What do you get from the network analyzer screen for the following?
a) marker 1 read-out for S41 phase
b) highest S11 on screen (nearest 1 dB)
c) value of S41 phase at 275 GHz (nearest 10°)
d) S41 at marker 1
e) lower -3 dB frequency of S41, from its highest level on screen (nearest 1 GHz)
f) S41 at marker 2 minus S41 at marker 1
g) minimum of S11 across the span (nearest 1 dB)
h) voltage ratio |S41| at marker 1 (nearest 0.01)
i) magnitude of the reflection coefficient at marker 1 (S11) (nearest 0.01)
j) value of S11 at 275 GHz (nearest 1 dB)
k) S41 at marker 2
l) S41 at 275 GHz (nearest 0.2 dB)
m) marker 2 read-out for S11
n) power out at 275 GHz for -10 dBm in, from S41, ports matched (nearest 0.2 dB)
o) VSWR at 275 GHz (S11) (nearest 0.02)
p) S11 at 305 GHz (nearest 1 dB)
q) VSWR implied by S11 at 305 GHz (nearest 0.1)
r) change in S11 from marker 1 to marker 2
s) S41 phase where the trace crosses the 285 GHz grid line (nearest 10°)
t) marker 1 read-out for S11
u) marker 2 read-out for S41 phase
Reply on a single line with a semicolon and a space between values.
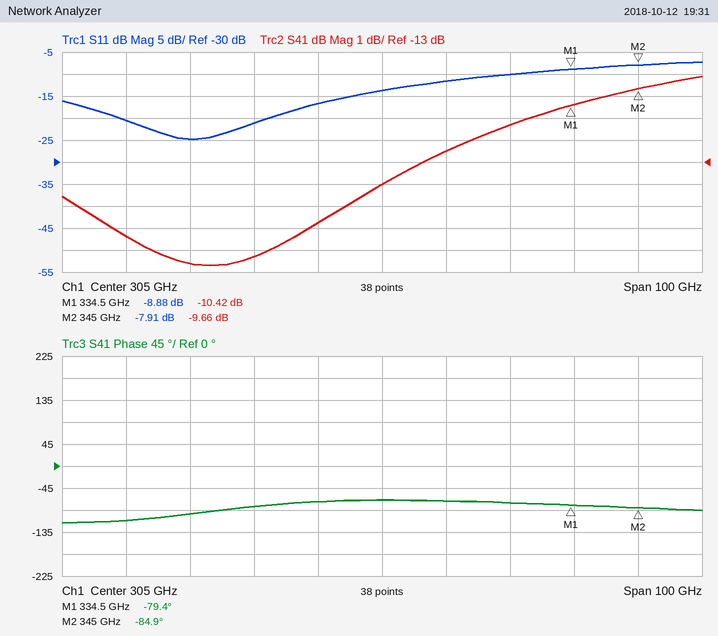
-79.4°; -7 dB; -100°; -10.42 dB; 318 GHz; 0.76 dB; -25 dB; 0.30; 0.36; -25 dB; -9.66 dB; -17.6 dB; -7.91 dB; -27.6 dBm; 1.12; -14 dB; 1.5; 0.97 dB; -80°; -8.88 dB; -84.9°
